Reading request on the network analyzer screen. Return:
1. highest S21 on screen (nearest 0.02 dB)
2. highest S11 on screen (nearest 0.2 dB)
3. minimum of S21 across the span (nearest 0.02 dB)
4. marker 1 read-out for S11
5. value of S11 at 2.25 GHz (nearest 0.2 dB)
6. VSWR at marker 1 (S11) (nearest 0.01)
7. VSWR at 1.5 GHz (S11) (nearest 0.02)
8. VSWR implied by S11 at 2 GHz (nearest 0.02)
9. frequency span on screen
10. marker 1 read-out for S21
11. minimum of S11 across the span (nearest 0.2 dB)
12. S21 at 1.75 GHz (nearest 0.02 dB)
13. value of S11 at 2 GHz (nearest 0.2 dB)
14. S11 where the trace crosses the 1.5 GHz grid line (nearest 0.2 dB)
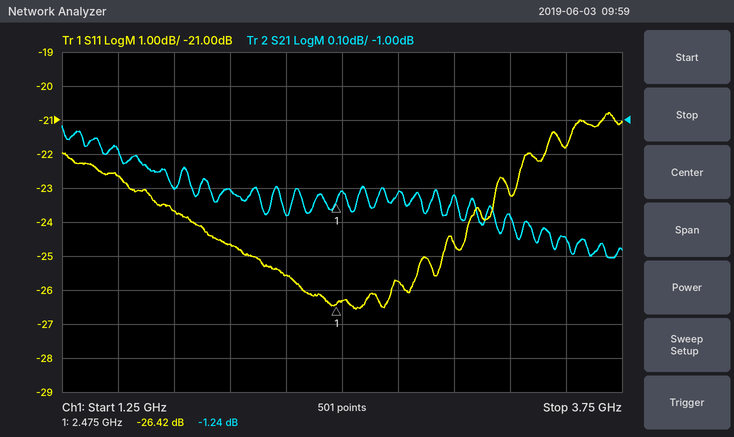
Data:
-1.02 dB
-20.8 dB
-1.40 dB
-26.42 dB
-25.6 dB
1.10
1.16
1.12
2.5 GHz
-1.24 dB
-26.6 dB
-1.20 dB
-24.6 dB
-22.6 dB
